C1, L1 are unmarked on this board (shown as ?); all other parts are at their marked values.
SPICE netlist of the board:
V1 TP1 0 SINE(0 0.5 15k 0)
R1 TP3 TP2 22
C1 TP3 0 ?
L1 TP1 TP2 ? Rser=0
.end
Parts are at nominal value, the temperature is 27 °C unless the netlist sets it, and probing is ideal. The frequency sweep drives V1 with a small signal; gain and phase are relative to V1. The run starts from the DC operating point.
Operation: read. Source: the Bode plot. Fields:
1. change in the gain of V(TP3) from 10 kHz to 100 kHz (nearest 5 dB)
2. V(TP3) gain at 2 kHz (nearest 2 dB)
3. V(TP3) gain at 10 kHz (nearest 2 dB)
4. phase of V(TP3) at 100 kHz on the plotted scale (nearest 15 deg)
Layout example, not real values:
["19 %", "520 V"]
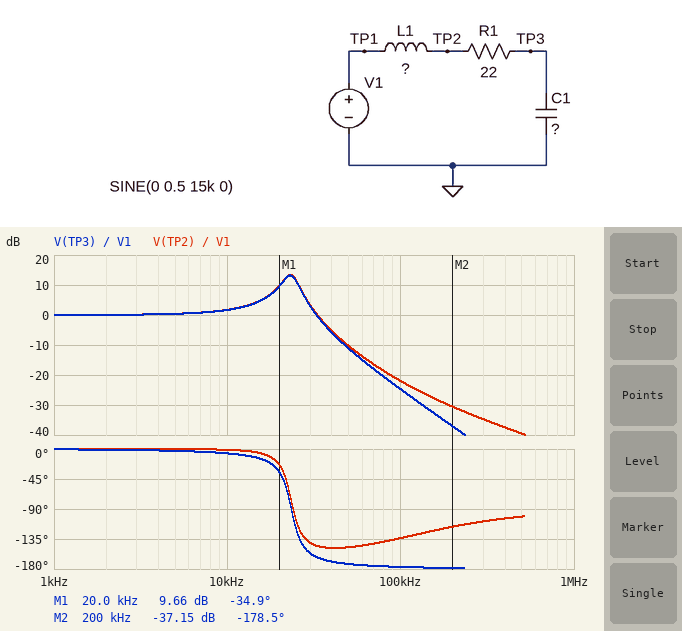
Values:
["-25 dB", "0 dB", "2 dB", "-180 deg"]
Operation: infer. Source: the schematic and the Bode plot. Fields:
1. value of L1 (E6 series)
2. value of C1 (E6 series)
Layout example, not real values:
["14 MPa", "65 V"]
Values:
["680 µH", "68 nF"]
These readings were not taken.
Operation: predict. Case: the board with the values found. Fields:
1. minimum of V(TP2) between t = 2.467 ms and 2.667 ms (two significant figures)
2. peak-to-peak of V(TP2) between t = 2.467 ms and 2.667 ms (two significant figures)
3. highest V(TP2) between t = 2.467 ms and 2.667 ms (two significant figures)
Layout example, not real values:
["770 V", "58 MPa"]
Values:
["-830 mV", "1.7 V", "830 mV"]
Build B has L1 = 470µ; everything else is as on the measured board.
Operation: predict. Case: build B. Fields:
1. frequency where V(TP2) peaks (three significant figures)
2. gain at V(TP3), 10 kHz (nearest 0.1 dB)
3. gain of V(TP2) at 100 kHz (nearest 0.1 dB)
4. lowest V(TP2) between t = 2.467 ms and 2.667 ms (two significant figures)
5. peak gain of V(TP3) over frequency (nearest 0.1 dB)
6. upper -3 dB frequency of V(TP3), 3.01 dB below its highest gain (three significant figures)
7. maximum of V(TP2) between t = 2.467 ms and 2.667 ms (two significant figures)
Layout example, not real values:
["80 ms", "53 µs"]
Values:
["27.7 kHz", "1.1 dB", "-18.6 dB", "-690 mV", "11.6 dB", "31.2 kHz", "690 mV"]
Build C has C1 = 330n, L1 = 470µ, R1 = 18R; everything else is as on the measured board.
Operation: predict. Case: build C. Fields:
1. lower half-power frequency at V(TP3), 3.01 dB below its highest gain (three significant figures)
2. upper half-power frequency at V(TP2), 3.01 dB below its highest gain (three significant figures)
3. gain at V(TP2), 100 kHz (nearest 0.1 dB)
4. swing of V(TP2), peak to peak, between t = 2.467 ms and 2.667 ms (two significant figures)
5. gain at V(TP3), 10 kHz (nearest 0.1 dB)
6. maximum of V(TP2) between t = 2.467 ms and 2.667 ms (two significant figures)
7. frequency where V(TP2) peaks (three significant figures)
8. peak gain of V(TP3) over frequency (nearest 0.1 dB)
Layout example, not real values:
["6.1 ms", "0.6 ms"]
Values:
["8.31 kHz", "15.1 kHz", "-23.9 dB", "1.7 V", "5.4 dB", "850 mV", "12.2 kHz", "6.7 dB"]
